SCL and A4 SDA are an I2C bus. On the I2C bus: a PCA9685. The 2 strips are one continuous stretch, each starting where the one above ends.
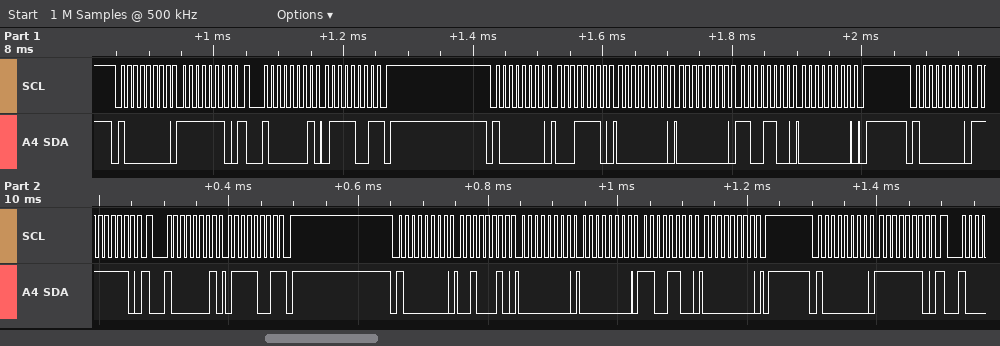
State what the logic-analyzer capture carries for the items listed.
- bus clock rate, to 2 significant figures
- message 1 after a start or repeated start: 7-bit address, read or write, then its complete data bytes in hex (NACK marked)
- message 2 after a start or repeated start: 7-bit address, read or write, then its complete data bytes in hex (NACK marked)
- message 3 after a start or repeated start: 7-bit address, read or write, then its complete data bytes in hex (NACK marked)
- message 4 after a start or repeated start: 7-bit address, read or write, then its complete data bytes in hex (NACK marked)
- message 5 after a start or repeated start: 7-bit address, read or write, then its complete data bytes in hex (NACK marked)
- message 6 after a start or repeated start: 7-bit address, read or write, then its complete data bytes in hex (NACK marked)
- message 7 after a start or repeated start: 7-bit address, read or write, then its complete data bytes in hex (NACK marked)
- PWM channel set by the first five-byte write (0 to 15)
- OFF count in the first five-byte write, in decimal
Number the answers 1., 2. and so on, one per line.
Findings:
1. 100 kHz
2. 0x40 write: FE
3. 0x40 read: 79 NACK
4. 0x40 write: 1E 00 00 CC 00
5. 0x40 write: FE
6. 0x40 read: 79 NACK
7. 0x40 write: 22 00 00 CC 00
8. 0x40 write: FE
9. 6
10. 204
